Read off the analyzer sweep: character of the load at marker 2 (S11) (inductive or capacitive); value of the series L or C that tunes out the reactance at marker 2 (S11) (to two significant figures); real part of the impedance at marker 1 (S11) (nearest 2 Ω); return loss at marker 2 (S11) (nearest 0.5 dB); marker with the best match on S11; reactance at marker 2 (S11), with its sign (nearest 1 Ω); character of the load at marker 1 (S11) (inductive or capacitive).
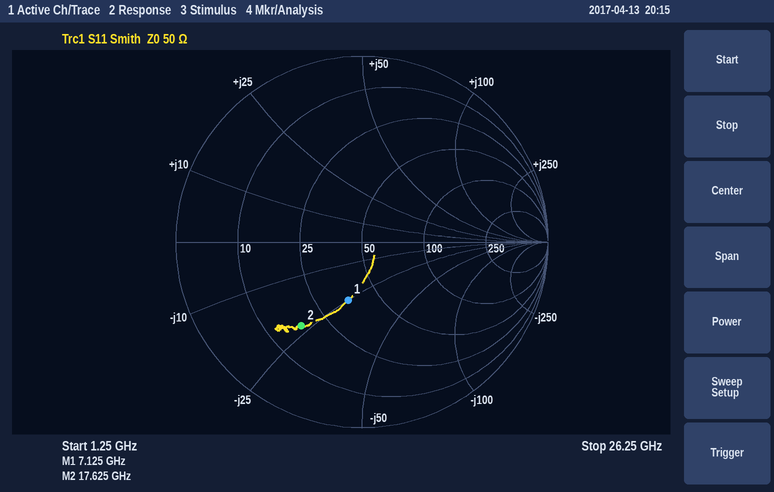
capacitive
210 pH
36 Ω
5.0 dB
marker 1
-23 Ω
capacitive
